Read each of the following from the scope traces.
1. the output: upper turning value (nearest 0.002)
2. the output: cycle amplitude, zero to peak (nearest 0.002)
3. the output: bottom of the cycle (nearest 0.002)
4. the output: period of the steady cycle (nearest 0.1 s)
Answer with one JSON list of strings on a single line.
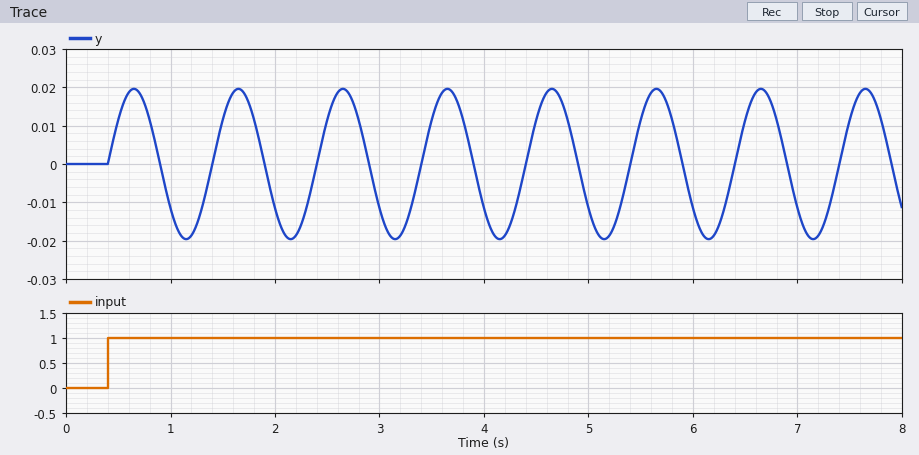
["0.020", "0.020", "-0.020", "1.0 s"]
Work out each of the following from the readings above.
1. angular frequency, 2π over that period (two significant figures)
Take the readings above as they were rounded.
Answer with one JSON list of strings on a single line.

["6.3 rad/s"]
